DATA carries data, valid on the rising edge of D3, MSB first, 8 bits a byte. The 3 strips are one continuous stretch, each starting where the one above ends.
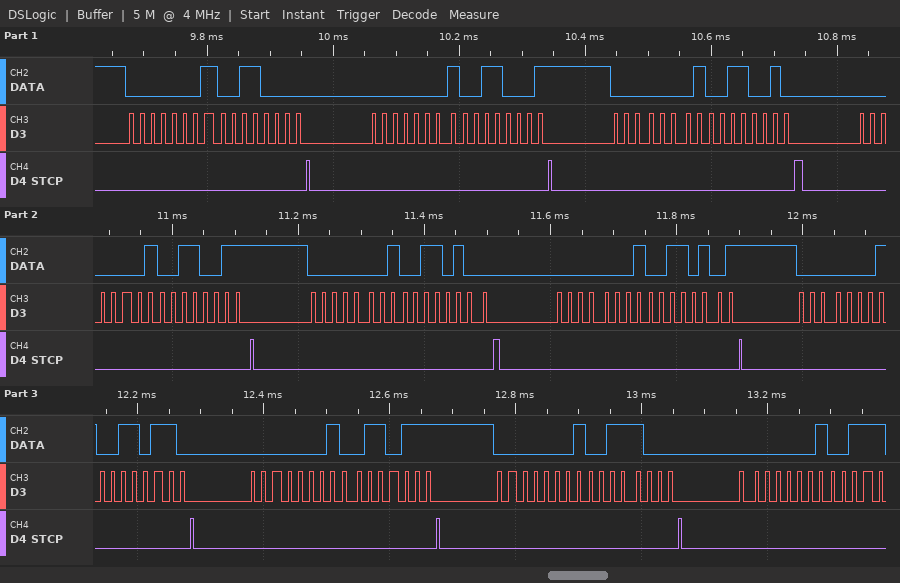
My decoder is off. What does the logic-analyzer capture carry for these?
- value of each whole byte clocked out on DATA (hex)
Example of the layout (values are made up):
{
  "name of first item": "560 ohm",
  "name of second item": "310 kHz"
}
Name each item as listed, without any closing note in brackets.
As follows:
{
  "value of each whole byte clocked out on DATA": "01 30 01 31 01 32 01 33 01 34 01 35 01 36 01 37 01 38 01"
}
